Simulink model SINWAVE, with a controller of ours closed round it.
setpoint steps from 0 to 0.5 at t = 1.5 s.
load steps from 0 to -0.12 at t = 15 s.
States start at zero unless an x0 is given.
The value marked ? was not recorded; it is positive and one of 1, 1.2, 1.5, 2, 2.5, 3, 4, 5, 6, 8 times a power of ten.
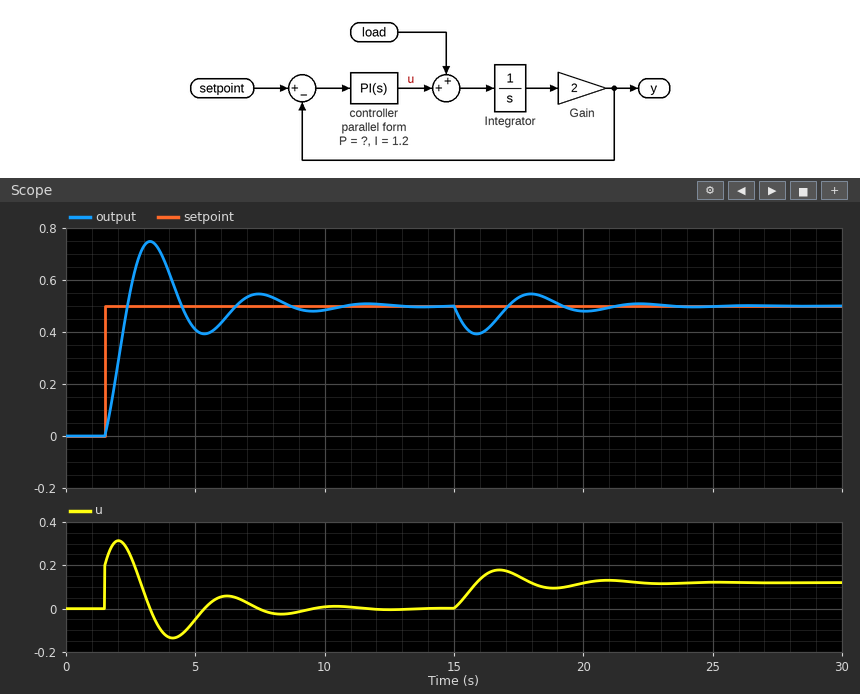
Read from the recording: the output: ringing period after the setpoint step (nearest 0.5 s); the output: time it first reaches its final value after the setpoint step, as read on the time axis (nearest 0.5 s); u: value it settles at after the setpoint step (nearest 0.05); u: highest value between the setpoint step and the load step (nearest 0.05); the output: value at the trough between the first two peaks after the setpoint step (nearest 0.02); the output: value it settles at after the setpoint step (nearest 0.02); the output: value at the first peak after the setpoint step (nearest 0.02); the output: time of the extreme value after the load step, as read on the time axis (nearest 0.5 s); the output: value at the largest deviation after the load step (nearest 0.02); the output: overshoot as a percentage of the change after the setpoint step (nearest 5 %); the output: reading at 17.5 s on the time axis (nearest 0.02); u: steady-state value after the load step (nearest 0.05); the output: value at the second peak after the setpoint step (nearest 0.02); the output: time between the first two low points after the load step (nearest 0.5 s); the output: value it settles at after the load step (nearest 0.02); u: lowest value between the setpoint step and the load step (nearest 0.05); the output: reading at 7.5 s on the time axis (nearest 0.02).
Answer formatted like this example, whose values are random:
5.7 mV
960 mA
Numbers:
4.0 s
2.5 s
0.00
0.30
0.40
0.50
0.74
16.0 s
0.40
50 %
0.54
0.10
0.54
4.0 s
0.50
-0.15
0.54
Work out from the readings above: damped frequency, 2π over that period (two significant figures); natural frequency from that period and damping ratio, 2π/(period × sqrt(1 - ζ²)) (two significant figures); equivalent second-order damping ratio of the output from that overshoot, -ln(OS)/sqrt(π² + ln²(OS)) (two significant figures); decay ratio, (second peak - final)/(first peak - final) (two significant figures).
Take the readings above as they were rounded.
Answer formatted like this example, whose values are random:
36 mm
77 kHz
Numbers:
1.6 rad/s
1.6 rad/s
0.22
0.17
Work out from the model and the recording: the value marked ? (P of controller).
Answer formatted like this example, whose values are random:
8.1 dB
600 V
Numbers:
0.4
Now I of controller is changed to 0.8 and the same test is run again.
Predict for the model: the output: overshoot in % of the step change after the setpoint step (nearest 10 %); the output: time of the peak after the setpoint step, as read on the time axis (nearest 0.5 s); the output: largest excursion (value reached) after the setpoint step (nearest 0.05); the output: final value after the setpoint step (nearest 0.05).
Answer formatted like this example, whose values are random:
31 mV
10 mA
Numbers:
40 %
3.5 s
0.70
0.50
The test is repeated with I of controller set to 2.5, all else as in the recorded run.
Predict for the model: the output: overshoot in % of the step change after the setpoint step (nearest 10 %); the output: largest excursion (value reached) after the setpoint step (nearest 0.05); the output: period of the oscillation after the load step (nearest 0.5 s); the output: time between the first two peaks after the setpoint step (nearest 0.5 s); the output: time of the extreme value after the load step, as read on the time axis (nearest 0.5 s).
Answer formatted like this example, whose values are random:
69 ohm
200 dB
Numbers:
60 %
0.80
3.0 s
3.0 s
15.5 s
